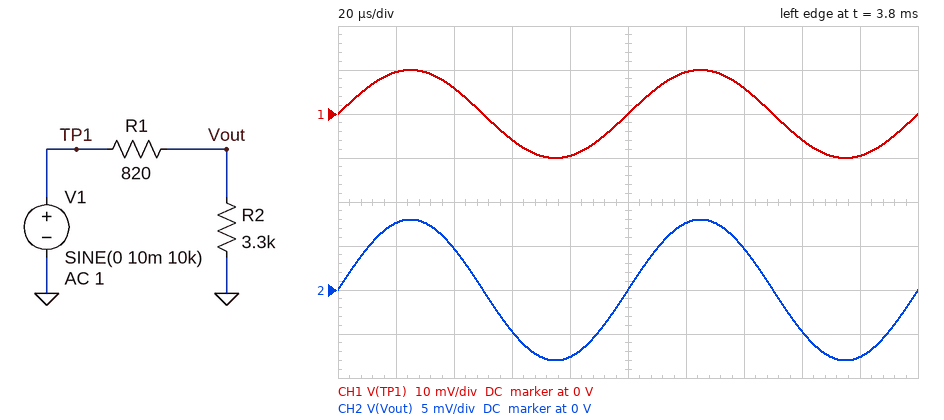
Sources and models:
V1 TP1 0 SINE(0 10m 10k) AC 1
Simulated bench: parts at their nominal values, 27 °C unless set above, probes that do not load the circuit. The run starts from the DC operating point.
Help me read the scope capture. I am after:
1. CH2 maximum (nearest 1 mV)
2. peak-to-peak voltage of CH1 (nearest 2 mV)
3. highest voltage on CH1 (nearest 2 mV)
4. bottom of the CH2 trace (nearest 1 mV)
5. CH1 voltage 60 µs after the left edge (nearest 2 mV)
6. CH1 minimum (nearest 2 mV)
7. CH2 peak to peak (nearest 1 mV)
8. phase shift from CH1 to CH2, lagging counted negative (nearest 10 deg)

8 mV
20 mV
10 mV
-8 mV
-6 mV
-10 mV
16 mV
0 deg
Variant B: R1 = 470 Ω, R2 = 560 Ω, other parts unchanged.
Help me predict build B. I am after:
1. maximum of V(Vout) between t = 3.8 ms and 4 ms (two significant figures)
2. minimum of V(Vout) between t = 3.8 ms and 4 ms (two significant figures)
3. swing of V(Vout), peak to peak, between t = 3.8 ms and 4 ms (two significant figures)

5.4 mV
-5.4 mV
11 mV
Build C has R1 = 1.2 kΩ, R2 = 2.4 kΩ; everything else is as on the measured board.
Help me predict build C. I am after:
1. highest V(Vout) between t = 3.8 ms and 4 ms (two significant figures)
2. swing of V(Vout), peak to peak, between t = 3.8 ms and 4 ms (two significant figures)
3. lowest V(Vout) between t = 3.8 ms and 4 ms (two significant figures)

6.7 mV
13 mV
-6.7 mV
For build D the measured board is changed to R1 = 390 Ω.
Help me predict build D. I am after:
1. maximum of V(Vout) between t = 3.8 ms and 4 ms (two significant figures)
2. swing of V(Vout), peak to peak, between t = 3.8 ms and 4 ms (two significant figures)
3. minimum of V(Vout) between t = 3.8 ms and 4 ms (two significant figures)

8.9 mV
18 mV
-8.9 mV
